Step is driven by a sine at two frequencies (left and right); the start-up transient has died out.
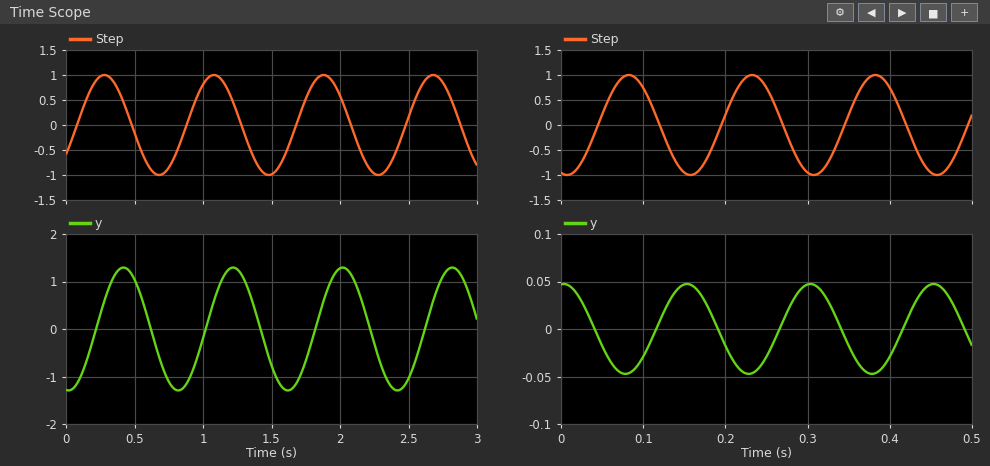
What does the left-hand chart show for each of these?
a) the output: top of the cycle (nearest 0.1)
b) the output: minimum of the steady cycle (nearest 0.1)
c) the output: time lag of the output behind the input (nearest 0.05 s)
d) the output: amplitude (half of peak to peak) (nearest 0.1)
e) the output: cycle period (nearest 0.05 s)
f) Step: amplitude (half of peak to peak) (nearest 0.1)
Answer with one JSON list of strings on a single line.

["1.3", "-1.3", "0.15 s", "1.3", "0.80 s", "1.0"]
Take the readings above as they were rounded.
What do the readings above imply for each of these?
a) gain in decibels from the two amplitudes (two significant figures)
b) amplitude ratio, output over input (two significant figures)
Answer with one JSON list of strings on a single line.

["2.3 dB", "1.3"]
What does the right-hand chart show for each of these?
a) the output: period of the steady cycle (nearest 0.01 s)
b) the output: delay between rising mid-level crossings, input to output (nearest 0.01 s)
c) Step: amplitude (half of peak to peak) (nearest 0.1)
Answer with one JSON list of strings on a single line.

["0.15 s", "0.07 s", "1.0"]
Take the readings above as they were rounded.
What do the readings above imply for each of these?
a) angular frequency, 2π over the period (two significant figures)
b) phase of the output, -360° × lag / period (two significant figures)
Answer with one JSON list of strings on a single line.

["42 rad/s", "-170°"]
